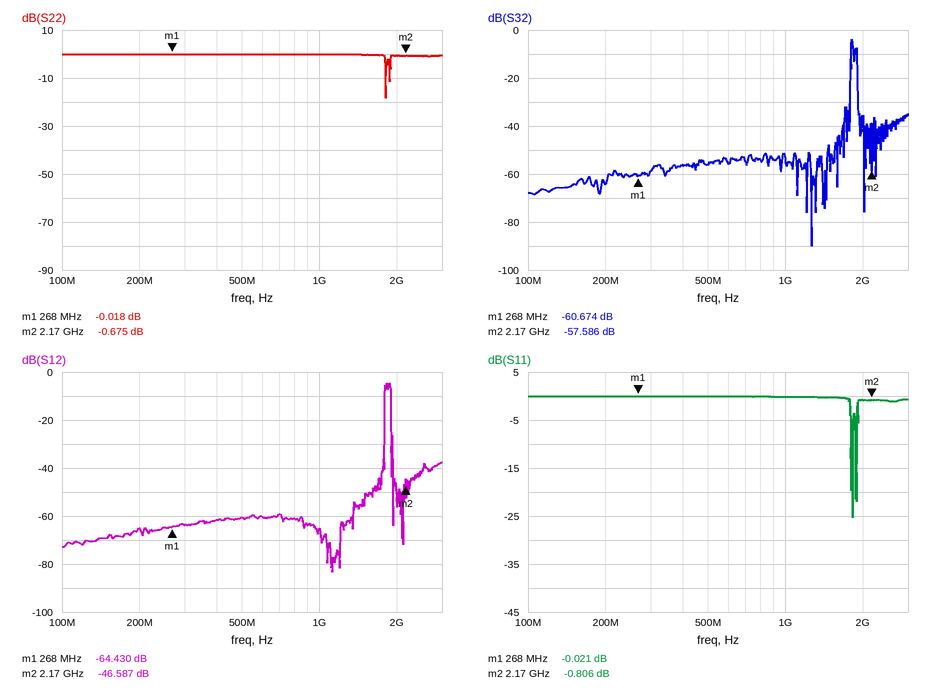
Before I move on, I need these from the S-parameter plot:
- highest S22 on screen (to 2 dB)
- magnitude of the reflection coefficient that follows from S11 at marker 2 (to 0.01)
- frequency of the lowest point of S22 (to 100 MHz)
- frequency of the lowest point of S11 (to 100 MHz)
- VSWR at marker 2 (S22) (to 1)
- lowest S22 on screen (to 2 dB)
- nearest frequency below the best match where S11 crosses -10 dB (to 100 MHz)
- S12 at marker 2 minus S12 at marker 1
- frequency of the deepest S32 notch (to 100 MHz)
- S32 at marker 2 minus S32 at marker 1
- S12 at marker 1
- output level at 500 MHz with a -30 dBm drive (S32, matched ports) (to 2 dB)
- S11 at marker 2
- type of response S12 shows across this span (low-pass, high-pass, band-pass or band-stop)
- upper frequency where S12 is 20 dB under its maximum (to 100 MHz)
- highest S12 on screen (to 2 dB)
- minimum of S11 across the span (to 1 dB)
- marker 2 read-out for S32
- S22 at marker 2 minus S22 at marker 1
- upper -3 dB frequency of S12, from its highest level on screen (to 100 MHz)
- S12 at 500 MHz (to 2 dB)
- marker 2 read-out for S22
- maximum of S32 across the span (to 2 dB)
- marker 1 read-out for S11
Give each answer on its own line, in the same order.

0 dB
0.91
1.8 GHz
1.8 GHz
26
-18 dB
1.8 GHz
17.843 dB
1.3 GHz
3.088 dB
-64.430 dB
-86 dBm
-0.806 dB
band-pass
1.9 GHz
-4 dB
-25 dB
-57.586 dB
-0.657 dB
1.9 GHz
-60 dB
-0.675 dB
-4 dB
-0.021 dB
